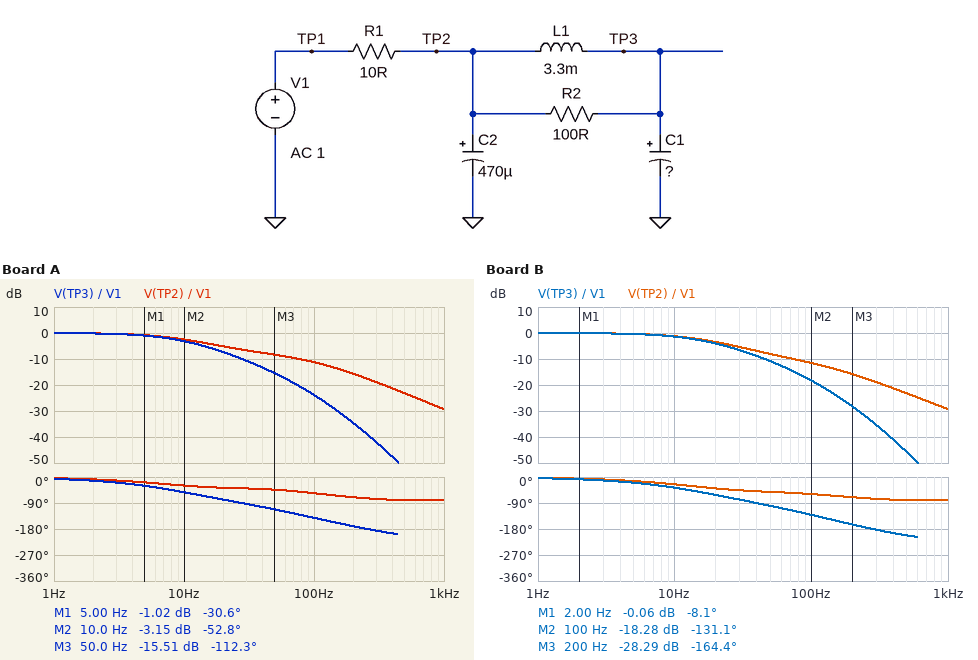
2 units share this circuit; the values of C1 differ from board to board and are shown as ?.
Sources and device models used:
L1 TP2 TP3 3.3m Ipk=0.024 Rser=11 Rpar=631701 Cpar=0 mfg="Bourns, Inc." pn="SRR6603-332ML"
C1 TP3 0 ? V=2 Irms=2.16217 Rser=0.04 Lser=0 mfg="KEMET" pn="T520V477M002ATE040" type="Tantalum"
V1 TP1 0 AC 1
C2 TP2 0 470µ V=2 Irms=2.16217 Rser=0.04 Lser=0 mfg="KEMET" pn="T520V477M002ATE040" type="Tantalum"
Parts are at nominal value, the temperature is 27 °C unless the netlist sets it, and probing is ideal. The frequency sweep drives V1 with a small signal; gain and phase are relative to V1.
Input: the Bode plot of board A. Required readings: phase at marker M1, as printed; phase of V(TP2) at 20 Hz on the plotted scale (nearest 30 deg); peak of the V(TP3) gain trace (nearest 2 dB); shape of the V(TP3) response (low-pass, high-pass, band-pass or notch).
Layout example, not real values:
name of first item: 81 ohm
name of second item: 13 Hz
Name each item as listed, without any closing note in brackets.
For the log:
phase at marker M1, as printed: -30.6 deg
phase of V(TP2) at 20 Hz on the plotted scale: -30 deg
peak of the V(TP3) gain trace: 0 dB
shape of the V(TP3) response: low-pass
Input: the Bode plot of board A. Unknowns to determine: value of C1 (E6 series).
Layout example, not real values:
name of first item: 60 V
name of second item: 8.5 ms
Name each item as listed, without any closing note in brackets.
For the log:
value of C1: 680 µF
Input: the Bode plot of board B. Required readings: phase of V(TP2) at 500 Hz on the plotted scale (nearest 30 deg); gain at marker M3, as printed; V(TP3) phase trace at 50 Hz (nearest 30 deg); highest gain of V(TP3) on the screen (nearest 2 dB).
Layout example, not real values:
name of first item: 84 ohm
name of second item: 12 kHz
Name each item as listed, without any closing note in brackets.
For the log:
phase of V(TP2) at 500 Hz on the plotted scale: -90 deg
gain at marker M3, as printed: -28.29 dB
V(TP3) phase trace at 50 Hz: -90 deg
highest gain of V(TP3) on the screen: 0 dB
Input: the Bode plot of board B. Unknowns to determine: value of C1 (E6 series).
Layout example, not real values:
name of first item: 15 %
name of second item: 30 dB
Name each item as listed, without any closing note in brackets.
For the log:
value of C1: 330 µF
